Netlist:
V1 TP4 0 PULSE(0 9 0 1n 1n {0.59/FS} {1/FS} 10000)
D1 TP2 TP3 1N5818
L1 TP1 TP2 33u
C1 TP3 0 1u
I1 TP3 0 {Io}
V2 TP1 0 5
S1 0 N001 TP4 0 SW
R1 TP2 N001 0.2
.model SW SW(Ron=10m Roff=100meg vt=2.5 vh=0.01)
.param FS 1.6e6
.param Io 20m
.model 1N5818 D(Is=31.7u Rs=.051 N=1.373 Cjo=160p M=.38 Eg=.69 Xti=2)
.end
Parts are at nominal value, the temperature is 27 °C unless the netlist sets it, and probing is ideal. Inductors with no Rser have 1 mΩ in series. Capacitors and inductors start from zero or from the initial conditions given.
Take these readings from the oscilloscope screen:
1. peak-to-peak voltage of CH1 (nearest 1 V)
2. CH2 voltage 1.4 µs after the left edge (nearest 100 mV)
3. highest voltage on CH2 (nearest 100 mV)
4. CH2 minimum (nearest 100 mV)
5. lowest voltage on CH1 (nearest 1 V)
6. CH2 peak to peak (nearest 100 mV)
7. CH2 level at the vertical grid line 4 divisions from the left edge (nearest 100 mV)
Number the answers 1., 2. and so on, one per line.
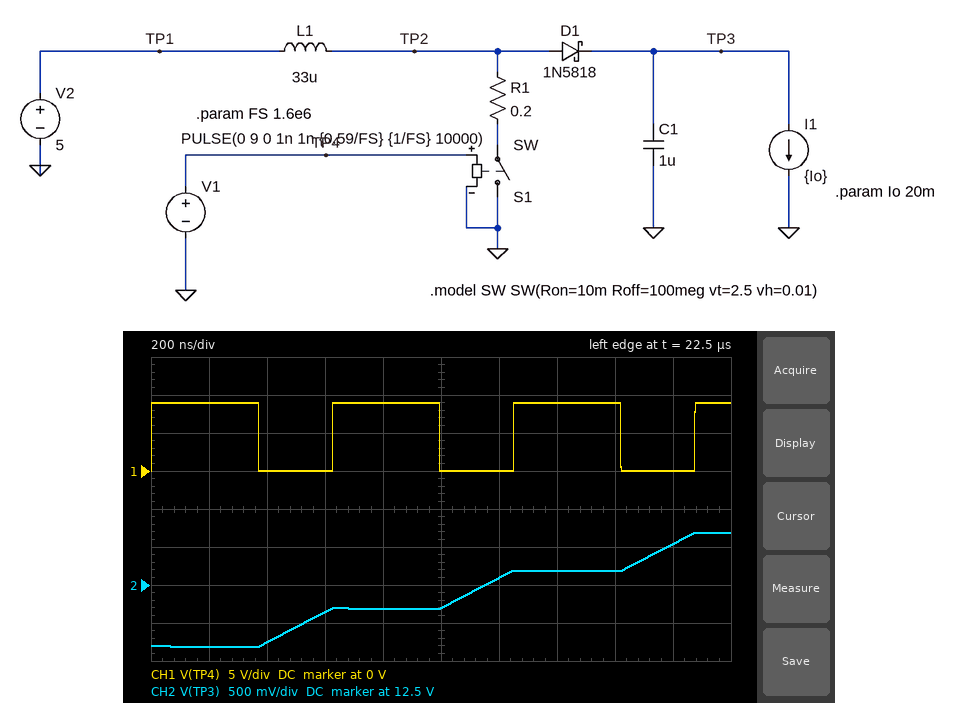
1. 9 V
2. 12.7 V
3. 13.2 V
4. 11.7 V
5. 0 V
6. 1.5 V
7. 12.2 V
